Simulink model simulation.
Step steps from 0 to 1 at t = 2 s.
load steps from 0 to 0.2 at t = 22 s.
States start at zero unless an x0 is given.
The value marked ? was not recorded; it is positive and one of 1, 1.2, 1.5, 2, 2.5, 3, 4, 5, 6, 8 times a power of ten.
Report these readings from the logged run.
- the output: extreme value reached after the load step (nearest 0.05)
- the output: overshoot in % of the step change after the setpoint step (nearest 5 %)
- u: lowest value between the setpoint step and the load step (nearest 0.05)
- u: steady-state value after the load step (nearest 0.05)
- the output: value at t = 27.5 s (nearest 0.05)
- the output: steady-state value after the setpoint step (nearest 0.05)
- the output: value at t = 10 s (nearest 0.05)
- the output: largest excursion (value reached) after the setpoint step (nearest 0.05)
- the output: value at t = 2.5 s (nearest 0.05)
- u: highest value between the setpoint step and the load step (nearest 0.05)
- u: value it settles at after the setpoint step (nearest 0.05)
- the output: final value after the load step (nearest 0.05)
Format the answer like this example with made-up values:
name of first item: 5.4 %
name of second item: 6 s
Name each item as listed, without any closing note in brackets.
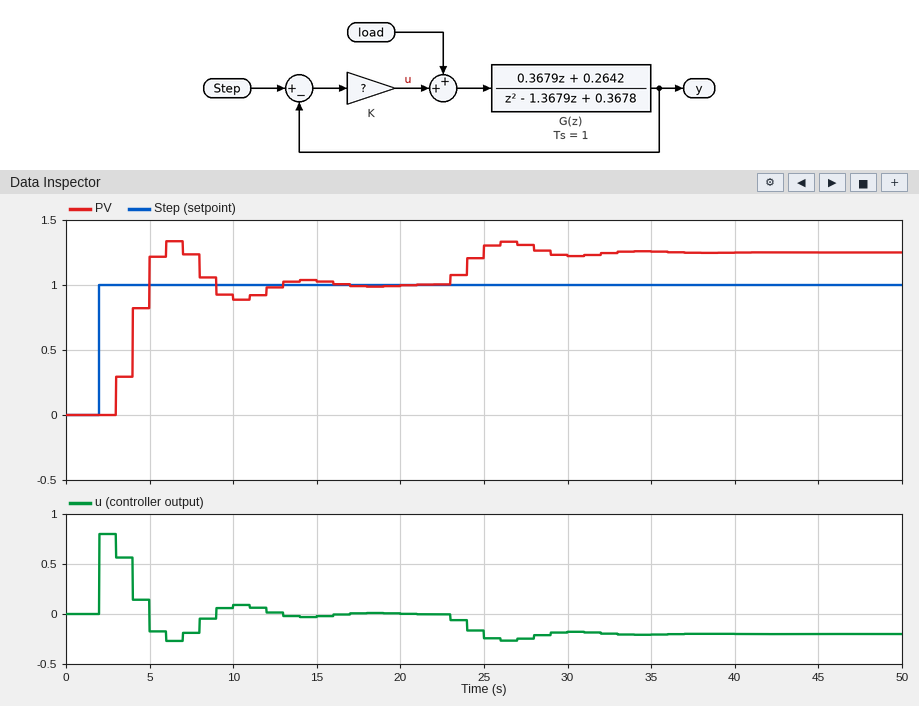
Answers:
the output: extreme value reached after the load step: 1.35
the output: overshoot in % of the step change after the setpoint step: 35 %
u: lowest value between the setpoint step and the load step: -0.25
u: steady-state value after the load step: -0.20
the output: value at t = 27.5 s: 1.30
the output: steady-state value after the setpoint step: 1.00
the output: value at t = 10 s: 0.90
the output: largest excursion (value reached) after the setpoint step: 1.35
the output: value at t = 2.5 s: 0.00
u: highest value between the setpoint step and the load step: 0.80
u: value it settles at after the setpoint step: 0.00
the output: final value after the load step: 1.25
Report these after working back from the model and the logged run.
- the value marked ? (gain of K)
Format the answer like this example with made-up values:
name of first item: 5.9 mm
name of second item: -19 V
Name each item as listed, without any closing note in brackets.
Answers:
the value marked ?: 0.8
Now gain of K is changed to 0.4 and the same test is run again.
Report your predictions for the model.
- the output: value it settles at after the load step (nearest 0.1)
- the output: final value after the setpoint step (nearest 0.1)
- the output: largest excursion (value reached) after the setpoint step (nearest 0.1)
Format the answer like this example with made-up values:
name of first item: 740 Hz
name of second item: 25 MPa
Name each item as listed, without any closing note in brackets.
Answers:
the output: value it settles at after the load step: 1.5
the output: final value after the setpoint step: 1.0
the output: largest excursion (value reached) after the setpoint step: 1.1
